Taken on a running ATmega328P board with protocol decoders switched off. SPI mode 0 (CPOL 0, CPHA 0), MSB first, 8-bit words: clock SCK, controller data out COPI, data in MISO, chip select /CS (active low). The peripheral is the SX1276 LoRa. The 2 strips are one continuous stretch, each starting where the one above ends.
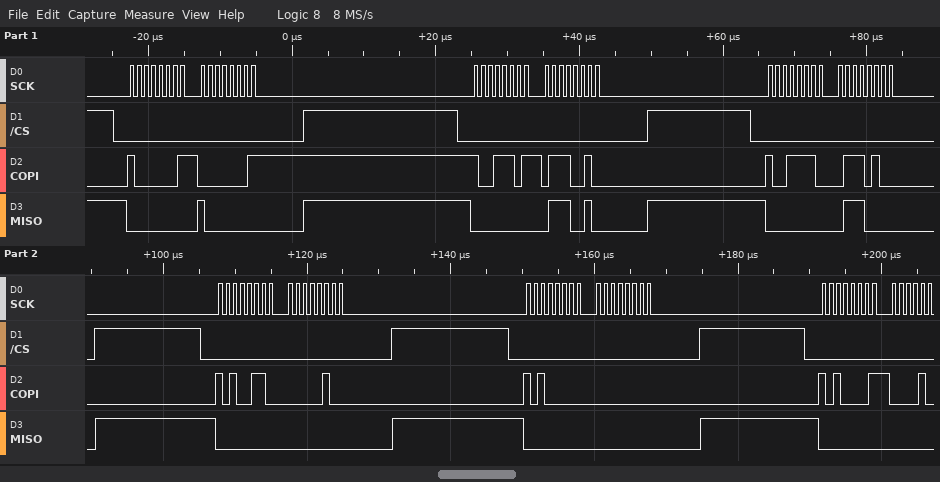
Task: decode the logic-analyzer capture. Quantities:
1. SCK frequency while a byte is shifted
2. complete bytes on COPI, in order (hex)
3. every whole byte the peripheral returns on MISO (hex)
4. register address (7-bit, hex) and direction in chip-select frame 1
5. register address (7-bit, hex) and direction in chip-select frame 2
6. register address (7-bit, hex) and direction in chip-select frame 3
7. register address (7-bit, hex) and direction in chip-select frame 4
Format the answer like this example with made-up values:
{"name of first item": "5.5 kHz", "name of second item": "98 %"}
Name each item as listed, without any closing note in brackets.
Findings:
{"SCK frequency while a byte is shifted": "1 MHz", "complete bytes on COPI, in order": "81 01 9D 72 9E 74 A6 04 A0 00 A1", "every whole byte the peripheral returns on MISO": "00 80 00 72 00 70 00 00 00 00 00", "register address (7-bit, hex) and direction in chip-select frame 1": "0x01 write", "register address (7-bit, hex) and direction in chip-select frame 2": "0x1D write", "register address (7-bit, hex) and direction in chip-select frame 3": "0x1E write", "register address (7-bit, hex) and direction in chip-select frame 4": "0x26 write"}
